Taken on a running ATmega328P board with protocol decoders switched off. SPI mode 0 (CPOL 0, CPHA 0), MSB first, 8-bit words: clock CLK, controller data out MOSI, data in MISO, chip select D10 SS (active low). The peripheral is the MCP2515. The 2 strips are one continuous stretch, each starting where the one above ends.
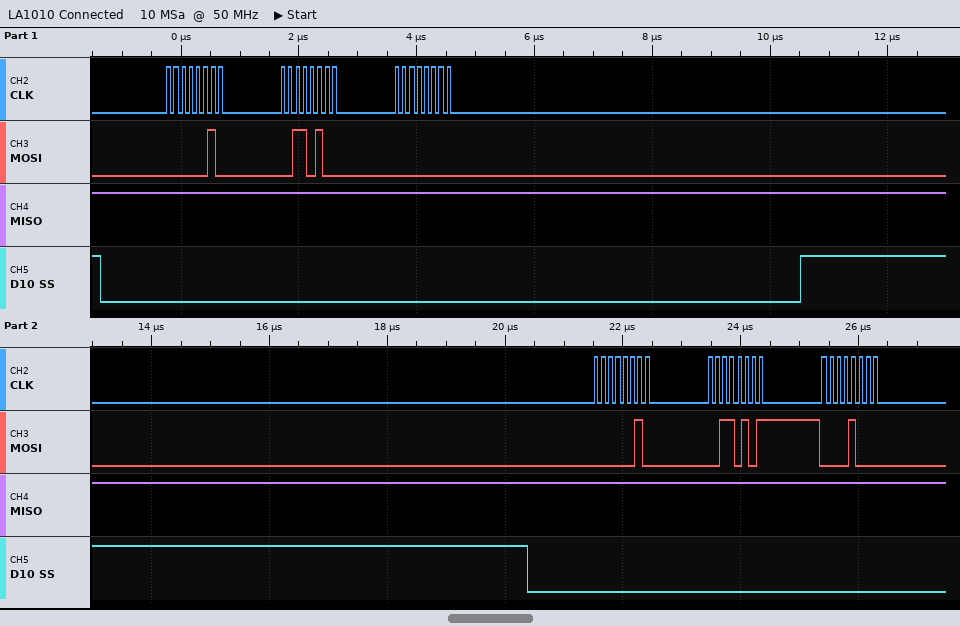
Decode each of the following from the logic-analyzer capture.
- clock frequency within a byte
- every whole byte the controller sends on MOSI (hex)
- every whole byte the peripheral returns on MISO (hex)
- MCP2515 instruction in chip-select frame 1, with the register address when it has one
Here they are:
8 MHz
02 34 00 02 35 08
FF FF FF FF FF FF
WRITE 0x34
